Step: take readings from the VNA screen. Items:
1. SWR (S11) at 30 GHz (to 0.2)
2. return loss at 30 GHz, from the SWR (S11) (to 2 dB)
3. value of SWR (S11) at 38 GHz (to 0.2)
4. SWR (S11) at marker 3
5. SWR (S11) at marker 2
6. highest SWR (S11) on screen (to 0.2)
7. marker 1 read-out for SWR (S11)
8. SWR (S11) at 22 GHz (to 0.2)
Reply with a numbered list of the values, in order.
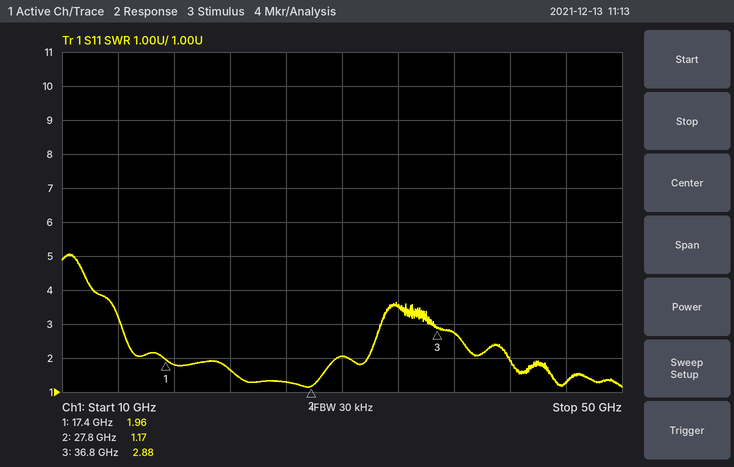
1. 2.0
2. 10 dB
3. 2.8
4. 2.88
5. 1.17
6. 5.0
7. 1.96
8. 1.6
